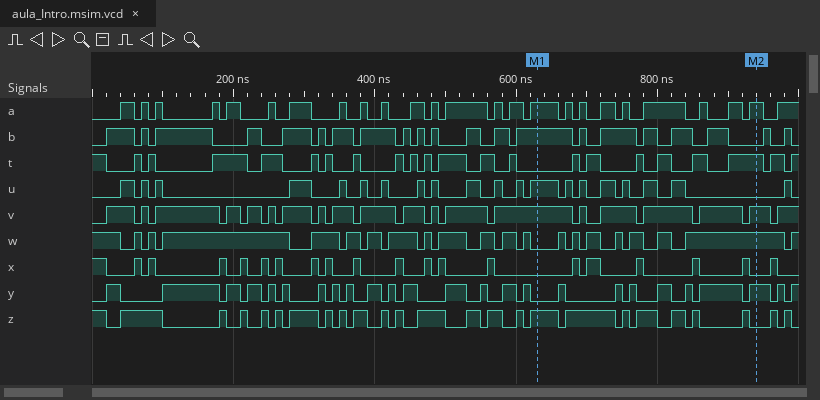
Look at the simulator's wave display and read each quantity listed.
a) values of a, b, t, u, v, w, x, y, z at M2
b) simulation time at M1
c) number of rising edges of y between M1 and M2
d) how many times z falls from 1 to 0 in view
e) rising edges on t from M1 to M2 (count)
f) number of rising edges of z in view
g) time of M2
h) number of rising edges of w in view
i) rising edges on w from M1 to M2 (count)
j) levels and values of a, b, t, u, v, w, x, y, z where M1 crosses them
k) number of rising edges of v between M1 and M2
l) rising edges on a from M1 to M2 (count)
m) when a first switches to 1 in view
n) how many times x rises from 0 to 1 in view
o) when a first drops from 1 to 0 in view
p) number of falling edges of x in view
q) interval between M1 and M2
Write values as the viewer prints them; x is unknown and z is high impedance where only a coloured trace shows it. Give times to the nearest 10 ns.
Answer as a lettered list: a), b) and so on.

a) a=1, b=0, t=1, u=0, v=1, w=1, x=0, y=1, z=0
b) 630 ns
c) 7
d) 25
e) 6
f) 24
g) 940 ns
h) 20
i) 7
j) a=1, b=1, t=0, u=1, v=1, w=0, x=0, y=0, z=1
k) 5
l) 8
m) 40 ns
n) 19
o) 60 ns
p) 20
q) 310 ns
